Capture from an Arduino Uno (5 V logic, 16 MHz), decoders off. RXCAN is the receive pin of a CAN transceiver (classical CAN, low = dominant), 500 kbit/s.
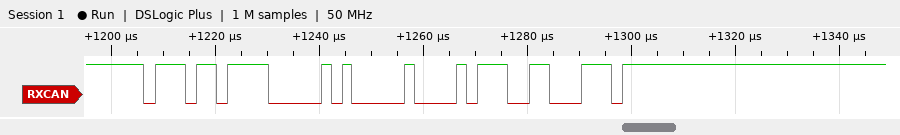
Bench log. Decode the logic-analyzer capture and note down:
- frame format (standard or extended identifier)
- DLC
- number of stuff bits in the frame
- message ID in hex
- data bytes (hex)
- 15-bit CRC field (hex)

standard
1
2
0x76F
00
0x2E63
